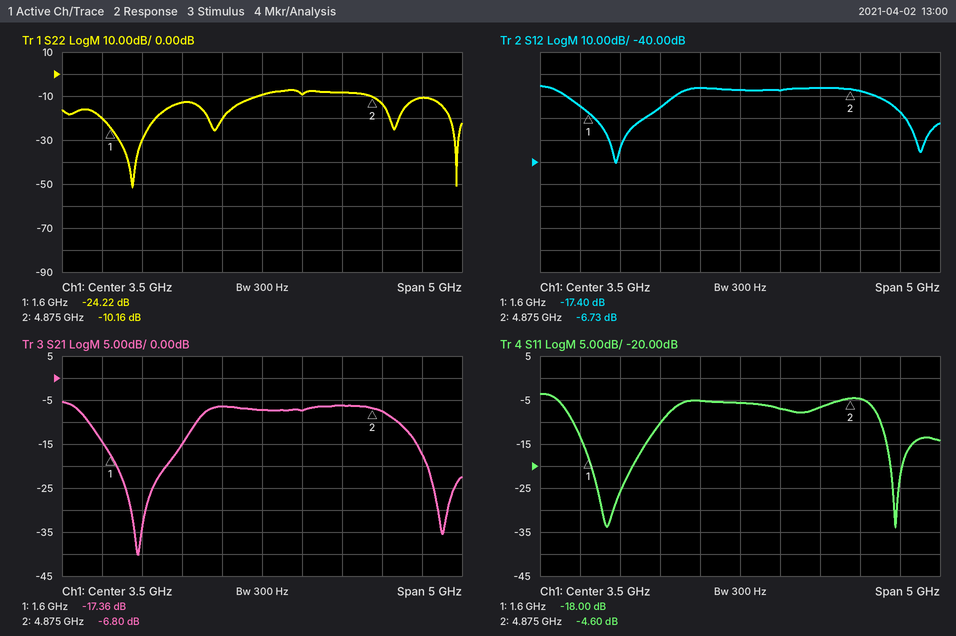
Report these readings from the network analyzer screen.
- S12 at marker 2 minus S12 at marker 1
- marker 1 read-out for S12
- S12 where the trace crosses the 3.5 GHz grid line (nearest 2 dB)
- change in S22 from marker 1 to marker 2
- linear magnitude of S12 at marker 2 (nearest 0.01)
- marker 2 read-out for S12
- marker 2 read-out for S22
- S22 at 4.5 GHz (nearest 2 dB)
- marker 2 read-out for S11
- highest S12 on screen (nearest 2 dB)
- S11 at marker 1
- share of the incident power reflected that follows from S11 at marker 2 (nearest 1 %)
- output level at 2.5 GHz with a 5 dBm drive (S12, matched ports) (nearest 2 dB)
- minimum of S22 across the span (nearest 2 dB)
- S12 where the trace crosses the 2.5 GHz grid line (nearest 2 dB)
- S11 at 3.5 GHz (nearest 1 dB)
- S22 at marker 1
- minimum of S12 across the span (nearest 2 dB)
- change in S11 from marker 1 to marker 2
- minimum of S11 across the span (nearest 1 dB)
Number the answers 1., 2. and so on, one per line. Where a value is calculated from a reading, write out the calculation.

1. -6.73 − (-17.4) = 10.67 dB
2. -17.40 dB
3. -8 dB
4. -10.16 − (-24.22) = 14.06 dB
5. 10^(-6.73/20) ≈ 0.46
6. -6.73 dB
7. -10.16 dB
8. -8 dB
9. -4.60 dB
10. -6 dB
11. -18.00 dB
12. 10^(-4.6/10) ≈ 35 %
13. 5 dBm + (-16 dB) = -10 dBm
14. -52 dB
15. -16 dB
16. -6 dB
17. -24.22 dB
18. -40 dB
19. -4.6 − (-18) = 13.40 dB
20. -34 dB
